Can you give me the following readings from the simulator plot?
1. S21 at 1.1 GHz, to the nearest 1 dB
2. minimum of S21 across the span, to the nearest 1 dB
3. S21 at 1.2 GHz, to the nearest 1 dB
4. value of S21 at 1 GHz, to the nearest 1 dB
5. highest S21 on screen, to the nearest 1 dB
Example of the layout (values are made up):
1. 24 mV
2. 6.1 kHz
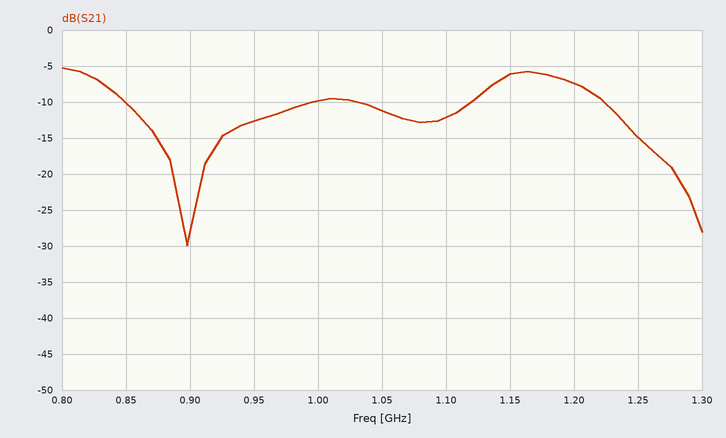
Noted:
1. -12 dB
2. -30 dB
3. -7 dB
4. -10 dB
5. -5 dB
